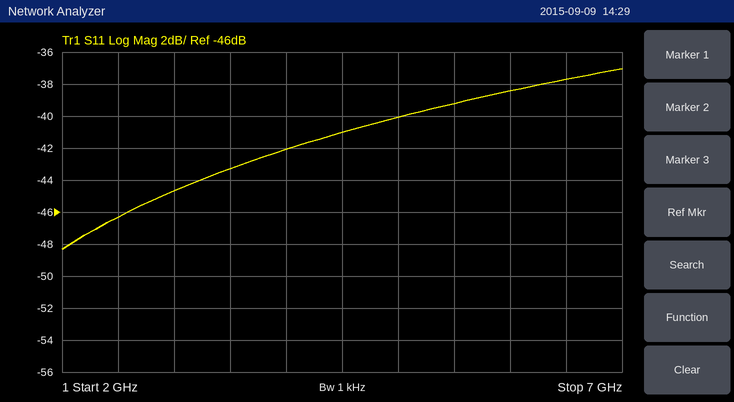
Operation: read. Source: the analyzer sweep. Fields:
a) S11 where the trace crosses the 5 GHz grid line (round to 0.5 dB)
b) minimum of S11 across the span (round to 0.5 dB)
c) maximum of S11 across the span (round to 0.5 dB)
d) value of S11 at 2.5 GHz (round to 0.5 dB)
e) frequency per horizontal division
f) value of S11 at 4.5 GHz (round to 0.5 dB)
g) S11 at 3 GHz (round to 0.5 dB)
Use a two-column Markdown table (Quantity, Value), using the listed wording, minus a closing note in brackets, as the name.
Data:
| Quantity | Value |
|---|---|
| S11 where the trace crosses the 5 GHz grid line | -40.0 dB |
| minimum of S11 across the span | -48.5 dB |
| maximum of S11 across the span | -37.0 dB |
| value of S11 at 2.5 GHz | -46.5 dB |
| frequency per horizontal division | 500 MHz |
| value of S11 at 4.5 GHz | -41.0 dB |
| S11 at 3 GHz | -44.5 dB |
